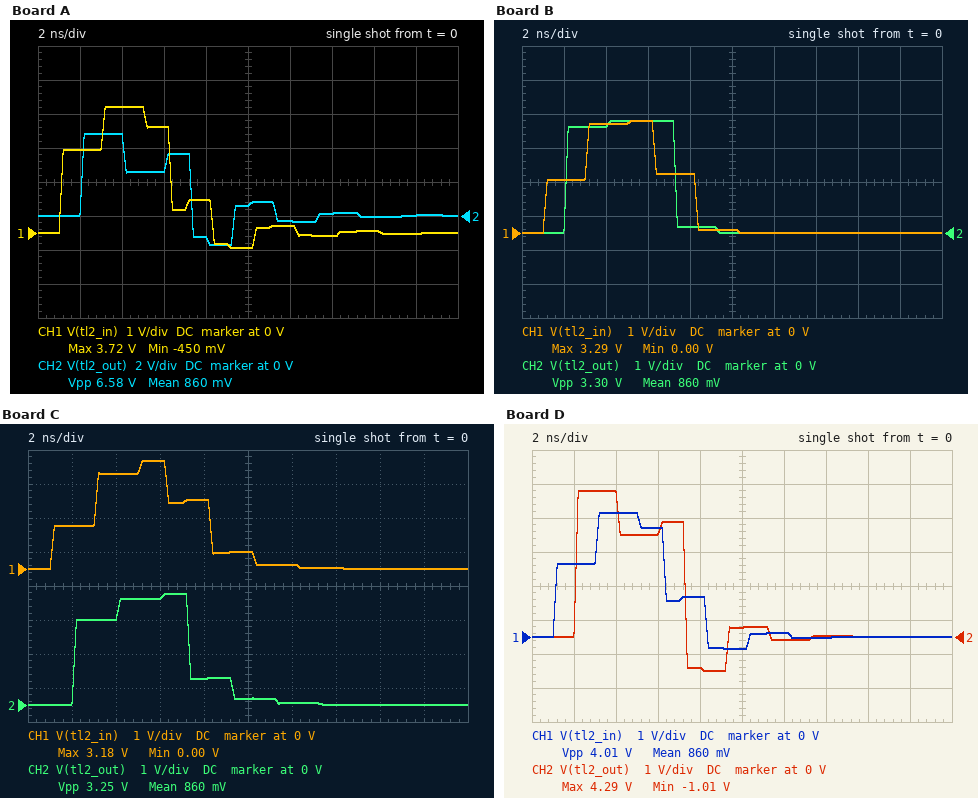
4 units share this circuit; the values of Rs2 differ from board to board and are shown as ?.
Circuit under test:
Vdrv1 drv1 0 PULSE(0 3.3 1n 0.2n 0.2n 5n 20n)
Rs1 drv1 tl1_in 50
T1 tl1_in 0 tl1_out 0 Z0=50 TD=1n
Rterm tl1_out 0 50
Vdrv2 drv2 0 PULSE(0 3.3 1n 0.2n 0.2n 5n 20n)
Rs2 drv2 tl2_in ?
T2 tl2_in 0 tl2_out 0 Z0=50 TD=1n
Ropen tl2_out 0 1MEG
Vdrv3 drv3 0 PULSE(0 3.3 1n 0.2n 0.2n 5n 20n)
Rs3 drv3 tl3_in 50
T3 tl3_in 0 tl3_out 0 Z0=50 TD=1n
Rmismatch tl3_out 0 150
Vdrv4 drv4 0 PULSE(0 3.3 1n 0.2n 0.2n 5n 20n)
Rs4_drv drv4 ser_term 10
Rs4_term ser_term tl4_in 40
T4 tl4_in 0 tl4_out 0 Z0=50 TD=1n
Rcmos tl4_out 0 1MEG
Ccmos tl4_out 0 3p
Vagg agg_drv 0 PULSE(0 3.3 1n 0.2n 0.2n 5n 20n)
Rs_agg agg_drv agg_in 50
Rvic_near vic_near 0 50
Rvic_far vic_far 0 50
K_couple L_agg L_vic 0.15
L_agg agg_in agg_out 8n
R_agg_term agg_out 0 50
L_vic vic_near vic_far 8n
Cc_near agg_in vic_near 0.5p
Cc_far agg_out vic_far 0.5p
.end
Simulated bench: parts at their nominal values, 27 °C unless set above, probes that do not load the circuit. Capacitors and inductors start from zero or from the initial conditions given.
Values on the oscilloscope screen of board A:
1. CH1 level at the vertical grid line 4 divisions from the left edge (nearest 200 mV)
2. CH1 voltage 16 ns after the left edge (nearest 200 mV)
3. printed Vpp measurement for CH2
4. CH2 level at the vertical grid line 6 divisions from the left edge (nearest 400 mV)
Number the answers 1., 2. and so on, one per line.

1. 1.0 V
2. 0 V
3. 6.58 V
4. -400 mV
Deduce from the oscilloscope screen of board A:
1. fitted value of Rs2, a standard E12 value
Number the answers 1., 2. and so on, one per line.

1. 18 Ω
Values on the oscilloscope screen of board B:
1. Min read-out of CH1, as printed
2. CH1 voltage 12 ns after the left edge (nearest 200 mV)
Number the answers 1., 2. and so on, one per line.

1. 0.00 V
2. 0 V
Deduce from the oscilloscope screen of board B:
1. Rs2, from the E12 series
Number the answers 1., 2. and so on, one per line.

1. 56 Ω
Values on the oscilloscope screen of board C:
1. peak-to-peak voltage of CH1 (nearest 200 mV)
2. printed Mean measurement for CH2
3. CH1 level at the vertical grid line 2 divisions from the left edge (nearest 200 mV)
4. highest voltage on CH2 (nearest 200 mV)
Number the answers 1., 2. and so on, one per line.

1. 3.2 V
2. 860 mV
3. 2.8 V
4. 3.2 V
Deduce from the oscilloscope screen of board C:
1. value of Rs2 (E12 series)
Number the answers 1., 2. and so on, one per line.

1. 82 Ω
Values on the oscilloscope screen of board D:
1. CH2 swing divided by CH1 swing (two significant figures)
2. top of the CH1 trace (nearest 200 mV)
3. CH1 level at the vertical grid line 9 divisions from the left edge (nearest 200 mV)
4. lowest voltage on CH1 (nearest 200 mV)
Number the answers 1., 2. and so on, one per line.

1. 1.3
2. 3.6 V
3. 0 V
4. -400 mV
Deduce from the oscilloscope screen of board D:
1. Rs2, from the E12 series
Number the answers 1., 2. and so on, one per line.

1. 27 Ω
